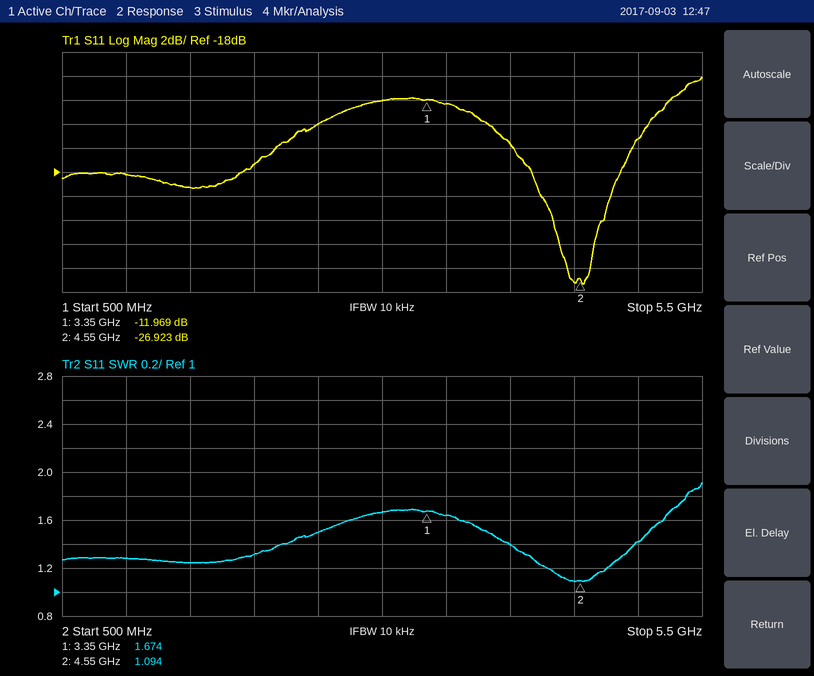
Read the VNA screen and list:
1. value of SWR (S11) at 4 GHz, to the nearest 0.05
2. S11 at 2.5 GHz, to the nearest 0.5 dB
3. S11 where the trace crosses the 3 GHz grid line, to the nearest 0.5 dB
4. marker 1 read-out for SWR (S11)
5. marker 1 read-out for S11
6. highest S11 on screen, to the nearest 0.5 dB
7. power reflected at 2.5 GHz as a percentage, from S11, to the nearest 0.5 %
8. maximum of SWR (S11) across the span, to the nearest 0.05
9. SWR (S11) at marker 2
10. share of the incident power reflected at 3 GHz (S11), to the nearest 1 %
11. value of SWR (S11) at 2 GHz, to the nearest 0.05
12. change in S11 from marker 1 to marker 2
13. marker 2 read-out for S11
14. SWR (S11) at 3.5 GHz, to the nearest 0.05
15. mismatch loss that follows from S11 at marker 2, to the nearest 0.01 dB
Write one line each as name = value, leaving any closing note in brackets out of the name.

value of SWR (S11) at 4 GHz, to the nearest 0.05 = 1.40
S11 at 2.5 GHz, to the nearest 0.5 dB = -14.0 dB
S11 where the trace crosses the 3 GHz grid line, to the nearest 0.5 dB = -12.0 dB
marker 1 read-out for SWR = 1.674
marker 1 read-out for S11 = -11.969 dB
highest S11 on screen, to the nearest 0.5 dB = -10.0 dB
power reflected at 2.5 GHz as a percentage, from S11, to the nearest 0.5 % = 4.0 %
maximum of SWR (S11) across the span, to the nearest 0.05 = 1.90
SWR (S11) at marker 2 = 1.094
share of the incident power reflected at 3 GHz (S11), to the nearest 1 % = 6 %
value of SWR (S11) at 2 GHz, to the nearest 0.05 = 1.30
change in S11 from marker 1 to marker 2 = -14.954 dB
marker 2 read-out for S11 = -26.923 dB
SWR (S11) at 3.5 GHz, to the nearest 0.05 = 1.65
mismatch loss that follows from S11 at marker 2, to the nearest 0.01 dB = 0.01 dB
